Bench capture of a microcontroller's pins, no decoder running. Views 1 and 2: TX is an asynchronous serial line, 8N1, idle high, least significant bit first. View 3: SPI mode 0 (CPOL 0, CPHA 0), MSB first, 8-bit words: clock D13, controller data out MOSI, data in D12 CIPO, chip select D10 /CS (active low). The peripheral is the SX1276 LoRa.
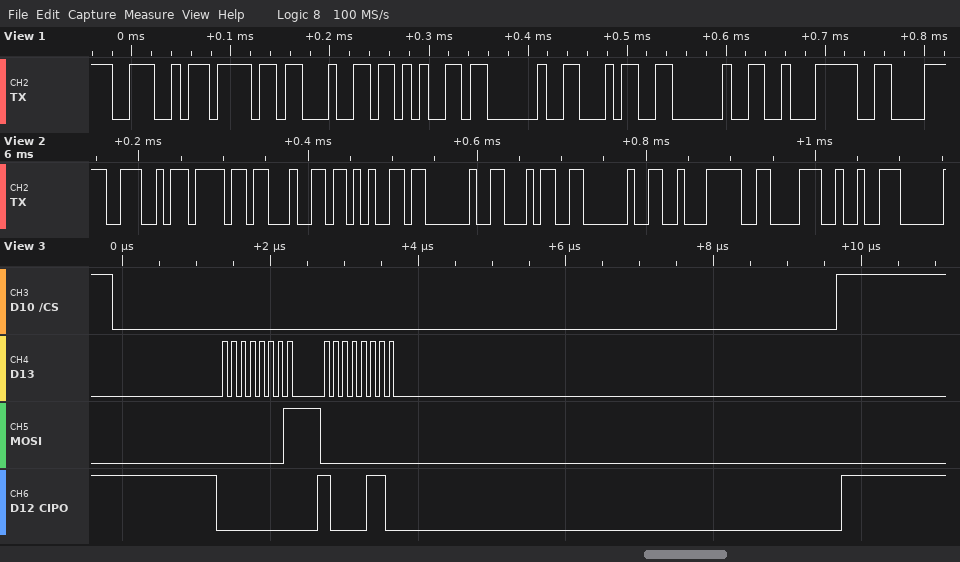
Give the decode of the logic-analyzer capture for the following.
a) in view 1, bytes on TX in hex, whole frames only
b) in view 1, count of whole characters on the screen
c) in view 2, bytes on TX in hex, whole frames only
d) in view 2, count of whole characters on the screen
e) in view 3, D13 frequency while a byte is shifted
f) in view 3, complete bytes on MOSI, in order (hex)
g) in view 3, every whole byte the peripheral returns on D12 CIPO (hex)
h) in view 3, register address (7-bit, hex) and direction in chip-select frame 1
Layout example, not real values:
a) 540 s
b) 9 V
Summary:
a) 0x4E 0x6F 0x64 0x65 0x20 0x34 0x20 0xE2 0x86
b) 9
c) 4E 6F 64 65 20 34 20 E2 86 92
d) 10
e) 8 MHz
f) 0x01 0x00
g) 0x00 0x86
h) 0x01 read
